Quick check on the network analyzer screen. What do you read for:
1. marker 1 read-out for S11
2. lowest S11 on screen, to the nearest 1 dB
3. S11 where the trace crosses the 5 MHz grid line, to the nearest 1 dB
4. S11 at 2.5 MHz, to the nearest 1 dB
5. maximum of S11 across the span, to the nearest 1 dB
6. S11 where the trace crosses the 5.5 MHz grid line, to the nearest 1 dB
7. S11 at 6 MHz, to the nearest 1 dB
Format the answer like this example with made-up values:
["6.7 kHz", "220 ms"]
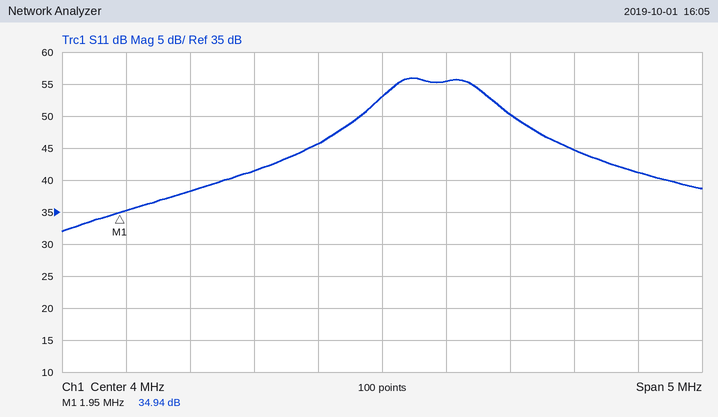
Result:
["34.94 dB", "32 dB", "50 dB", "38 dB", "56 dB", "45 dB", "41 dB"]
